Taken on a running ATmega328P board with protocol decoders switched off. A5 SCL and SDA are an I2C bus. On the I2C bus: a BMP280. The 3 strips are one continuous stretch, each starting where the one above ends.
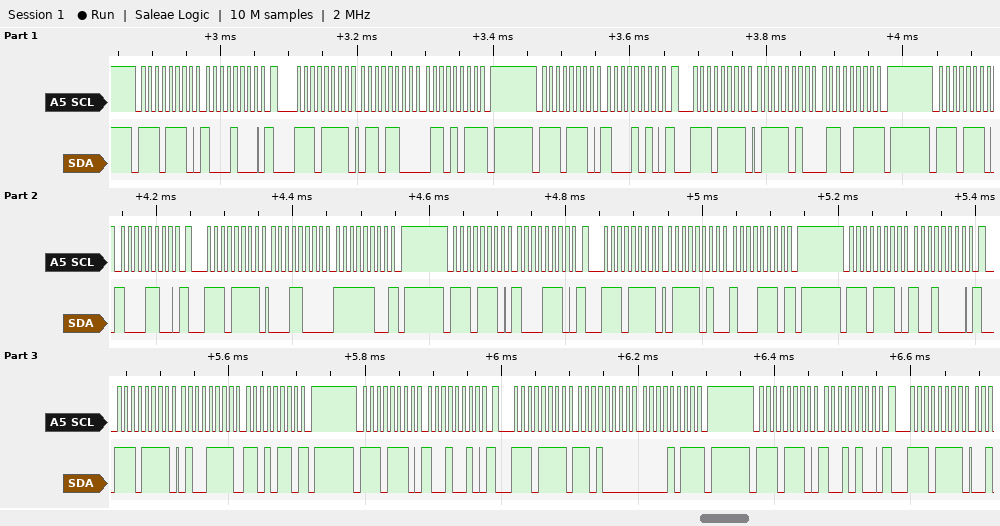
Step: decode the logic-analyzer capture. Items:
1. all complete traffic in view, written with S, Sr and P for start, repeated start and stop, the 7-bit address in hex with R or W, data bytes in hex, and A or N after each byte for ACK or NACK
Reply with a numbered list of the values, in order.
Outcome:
1. S 77W A 88 A Sr 77R A 6C A 6B N P S 77W A 8A A Sr 77R A 7A A 67 N P S 77W A 8C A Sr 77R A 18 A FC N P S 77W A 8E A Sr 77R A 7A A 8E N P S 77W A 90 A Sr 77R A 4F A D6 N P S 77W A 92 A Sr 77R A D0 A 0B N P S 77W A 94 A Sr 77R A
